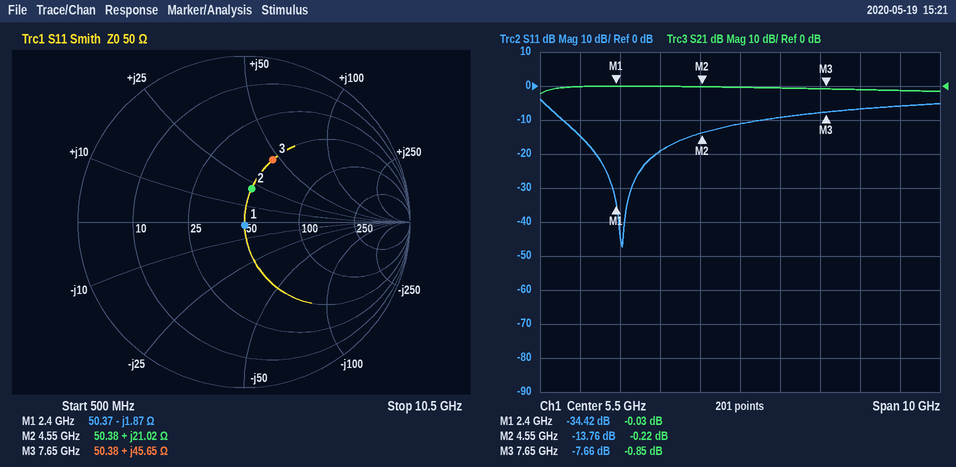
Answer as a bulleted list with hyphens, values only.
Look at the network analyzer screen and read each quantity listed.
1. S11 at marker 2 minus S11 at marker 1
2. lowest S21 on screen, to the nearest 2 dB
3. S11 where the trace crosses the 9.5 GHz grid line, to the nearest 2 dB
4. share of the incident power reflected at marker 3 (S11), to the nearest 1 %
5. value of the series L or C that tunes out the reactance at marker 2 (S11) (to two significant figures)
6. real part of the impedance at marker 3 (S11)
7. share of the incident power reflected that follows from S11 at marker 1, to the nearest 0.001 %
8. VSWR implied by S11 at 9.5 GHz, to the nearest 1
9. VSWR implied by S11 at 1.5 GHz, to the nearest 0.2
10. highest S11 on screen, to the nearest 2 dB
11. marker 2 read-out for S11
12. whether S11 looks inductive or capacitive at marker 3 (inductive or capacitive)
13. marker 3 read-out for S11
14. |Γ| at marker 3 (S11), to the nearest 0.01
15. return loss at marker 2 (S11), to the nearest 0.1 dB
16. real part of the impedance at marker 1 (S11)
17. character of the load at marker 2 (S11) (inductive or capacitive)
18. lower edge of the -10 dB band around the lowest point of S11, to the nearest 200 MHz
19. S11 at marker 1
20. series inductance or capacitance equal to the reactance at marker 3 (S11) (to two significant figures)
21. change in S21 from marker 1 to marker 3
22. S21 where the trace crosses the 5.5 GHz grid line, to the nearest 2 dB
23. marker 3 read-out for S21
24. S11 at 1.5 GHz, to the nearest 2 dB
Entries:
- 20.66 dB
- -2 dB
- -6 dB
- 17 %
- 1.7 pF
- 50.38 Ω
- 0.036 %
- 3
- 1.4
- -4 dB
- -13.76 dB
- inductive
- -7.66 dB
- 0.41
- 13.8 dB
- 50.37 Ω
- inductive
- 1.0 GHz
- -34.42 dB
- 950 pH
- -0.82 dB
- 0 dB
- -0.85 dB
- -14 dB
